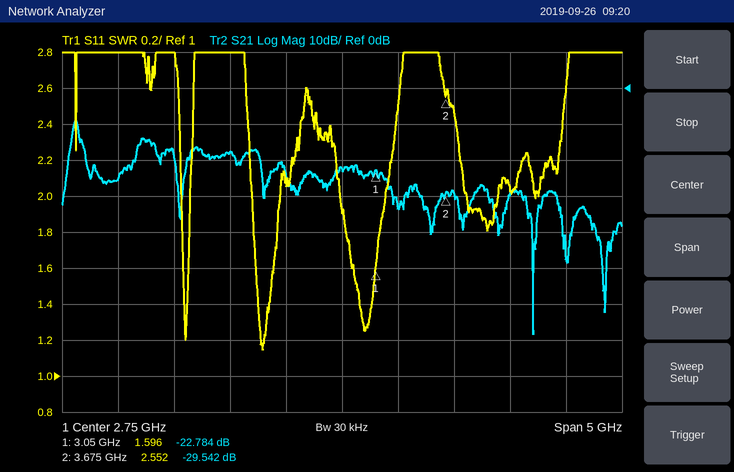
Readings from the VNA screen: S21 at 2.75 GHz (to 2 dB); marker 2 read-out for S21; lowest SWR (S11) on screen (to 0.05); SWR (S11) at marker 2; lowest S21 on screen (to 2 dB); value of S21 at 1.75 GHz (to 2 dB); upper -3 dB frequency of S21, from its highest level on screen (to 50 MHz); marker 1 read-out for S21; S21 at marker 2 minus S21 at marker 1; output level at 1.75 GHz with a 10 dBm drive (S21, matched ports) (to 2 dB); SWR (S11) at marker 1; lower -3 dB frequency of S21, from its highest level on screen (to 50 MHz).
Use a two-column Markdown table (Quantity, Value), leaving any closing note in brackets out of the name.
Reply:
| Quantity | Value |
|---|---|
| S21 at 2.75 GHz | -22 dB |
| marker 2 read-out for S21 | -29.542 dB |
| lowest SWR (S11) on screen | 1.15 |
| SWR (S11) at marker 2 | 2.552 |
| lowest S21 on screen | -68 dB |
| value of S21 at 1.75 GHz | -18 dB |
| upper -3 dB frequency of S21, from its highest level on screen | 400 MHz |
| marker 1 read-out for S21 | -22.784 dB |
| S21 at marker 2 minus S21 at marker 1 | -6.758 dB |
| output level at 1.75 GHz with a 10 dBm drive (S21, matched ports) | -8 dBm |
| SWR (S11) at marker 1 | 1.596 |
| lower -3 dB frequency of S21, from its highest level on screen | 350 MHz |
